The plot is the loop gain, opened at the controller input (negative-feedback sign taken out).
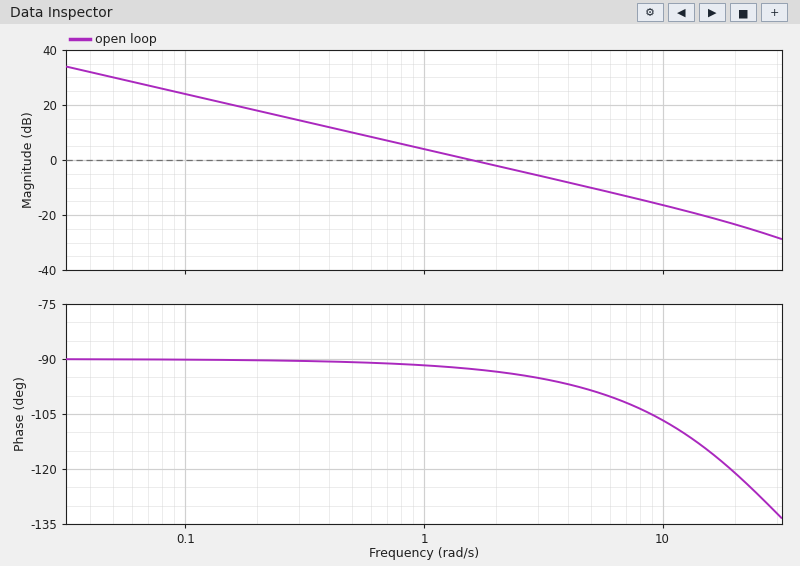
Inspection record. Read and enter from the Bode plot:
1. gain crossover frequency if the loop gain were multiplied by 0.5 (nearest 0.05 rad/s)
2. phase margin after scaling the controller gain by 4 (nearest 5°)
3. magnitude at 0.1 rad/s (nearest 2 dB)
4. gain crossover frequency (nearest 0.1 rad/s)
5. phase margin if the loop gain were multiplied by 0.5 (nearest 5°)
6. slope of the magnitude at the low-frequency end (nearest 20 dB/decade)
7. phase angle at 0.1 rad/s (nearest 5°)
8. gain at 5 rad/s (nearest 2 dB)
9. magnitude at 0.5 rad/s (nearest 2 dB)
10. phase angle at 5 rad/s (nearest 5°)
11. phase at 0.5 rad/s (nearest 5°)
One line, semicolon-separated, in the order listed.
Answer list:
0.80 rad/s; 80°; 24 dB; 1.6 rad/s; 90°; -20 dB/decade; -90°; -10 dB; 10 dB; -100°; -90°
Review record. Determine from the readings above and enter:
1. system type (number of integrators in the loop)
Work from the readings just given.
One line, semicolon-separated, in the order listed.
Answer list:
1
